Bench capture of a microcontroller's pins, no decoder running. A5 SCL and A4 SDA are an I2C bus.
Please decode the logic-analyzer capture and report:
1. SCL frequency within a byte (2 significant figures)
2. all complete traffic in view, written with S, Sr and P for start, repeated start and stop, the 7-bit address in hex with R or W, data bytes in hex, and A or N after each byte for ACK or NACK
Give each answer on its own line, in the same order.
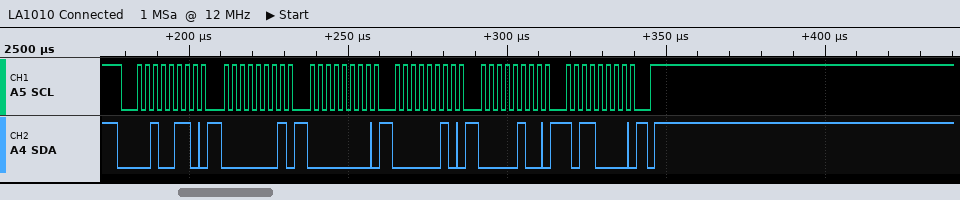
400 kHz
S 13W A 01 A 00 A 02 A 04 A B0 A P
